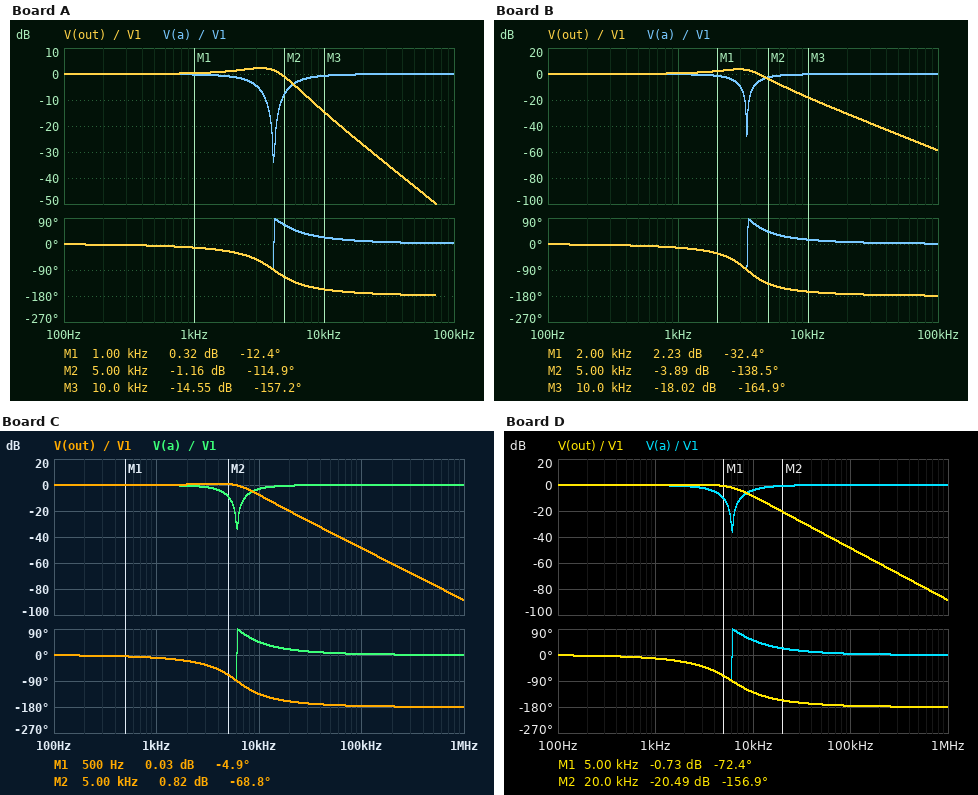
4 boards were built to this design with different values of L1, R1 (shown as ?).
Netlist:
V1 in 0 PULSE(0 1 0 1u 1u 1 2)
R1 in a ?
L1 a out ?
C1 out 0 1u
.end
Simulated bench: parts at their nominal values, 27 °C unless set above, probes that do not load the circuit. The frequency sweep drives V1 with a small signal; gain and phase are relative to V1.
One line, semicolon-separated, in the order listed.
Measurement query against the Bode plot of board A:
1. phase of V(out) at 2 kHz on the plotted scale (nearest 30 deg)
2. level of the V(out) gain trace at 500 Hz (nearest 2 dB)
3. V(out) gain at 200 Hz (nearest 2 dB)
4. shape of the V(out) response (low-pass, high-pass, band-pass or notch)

-30 deg; 0 dB; 0 dB; low-pass
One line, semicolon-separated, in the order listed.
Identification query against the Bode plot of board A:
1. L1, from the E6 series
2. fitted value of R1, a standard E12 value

1.5 mH; 33 Ω
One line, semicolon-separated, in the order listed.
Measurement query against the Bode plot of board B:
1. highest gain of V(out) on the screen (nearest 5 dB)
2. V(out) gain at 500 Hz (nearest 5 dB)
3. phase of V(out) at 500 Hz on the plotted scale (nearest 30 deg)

5 dB; 0 dB; 0 deg
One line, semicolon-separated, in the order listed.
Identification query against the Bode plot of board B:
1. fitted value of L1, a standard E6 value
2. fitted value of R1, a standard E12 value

2.2 mH; 33 Ω
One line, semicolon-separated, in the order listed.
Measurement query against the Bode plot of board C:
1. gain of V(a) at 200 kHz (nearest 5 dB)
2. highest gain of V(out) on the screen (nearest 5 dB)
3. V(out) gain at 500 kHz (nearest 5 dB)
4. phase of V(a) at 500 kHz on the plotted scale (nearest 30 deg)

0 dB; 0 dB; -75 dB; 0 deg
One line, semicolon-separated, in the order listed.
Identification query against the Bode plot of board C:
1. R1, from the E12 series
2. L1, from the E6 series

27 Ω; 680 µH
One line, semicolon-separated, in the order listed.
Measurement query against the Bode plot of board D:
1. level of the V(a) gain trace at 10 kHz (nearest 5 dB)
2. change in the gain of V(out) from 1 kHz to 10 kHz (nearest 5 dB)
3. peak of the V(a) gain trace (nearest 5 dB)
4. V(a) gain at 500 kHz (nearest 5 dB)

-5 dB; -10 dB; 0 dB; 0 dB
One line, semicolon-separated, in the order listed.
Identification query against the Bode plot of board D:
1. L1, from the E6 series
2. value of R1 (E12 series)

680 µH; 33 Ω
